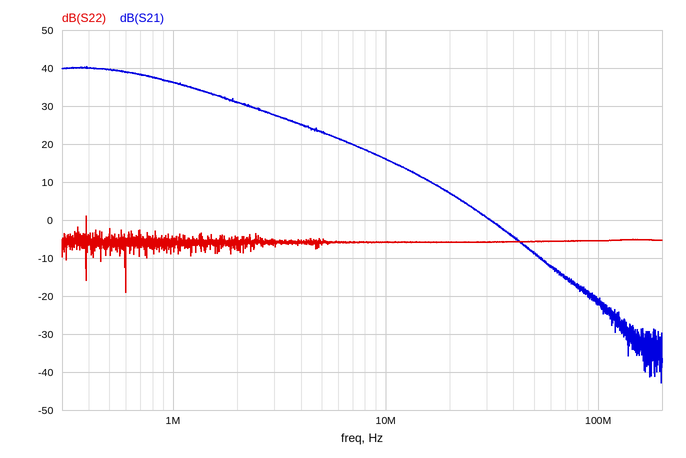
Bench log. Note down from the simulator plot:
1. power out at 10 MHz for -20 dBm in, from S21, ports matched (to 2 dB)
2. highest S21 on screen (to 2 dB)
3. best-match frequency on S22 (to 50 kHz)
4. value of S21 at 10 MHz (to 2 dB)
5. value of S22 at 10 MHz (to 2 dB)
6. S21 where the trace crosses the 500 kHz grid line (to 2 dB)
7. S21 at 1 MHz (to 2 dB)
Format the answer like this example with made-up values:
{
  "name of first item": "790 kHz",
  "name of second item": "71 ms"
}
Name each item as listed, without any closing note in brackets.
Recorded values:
{
  "power out at 10 MHz for -20 dBm in, from S21, ports matched": "-4 dBm",
  "highest S21 on screen": "40 dB",
  "best-match frequency on S22": "600 kHz",
  "value of S21 at 10 MHz": "16 dB",
  "value of S22 at 10 MHz": "-6 dB",
  "S21 where the trace crosses the 500 kHz grid line": "40 dB",
  "S21 at 1 MHz": "36 dB"
}
